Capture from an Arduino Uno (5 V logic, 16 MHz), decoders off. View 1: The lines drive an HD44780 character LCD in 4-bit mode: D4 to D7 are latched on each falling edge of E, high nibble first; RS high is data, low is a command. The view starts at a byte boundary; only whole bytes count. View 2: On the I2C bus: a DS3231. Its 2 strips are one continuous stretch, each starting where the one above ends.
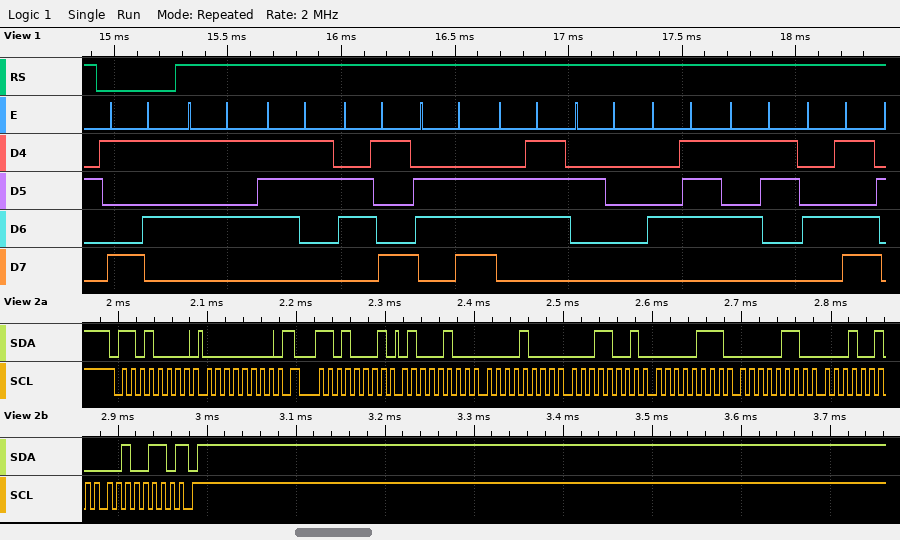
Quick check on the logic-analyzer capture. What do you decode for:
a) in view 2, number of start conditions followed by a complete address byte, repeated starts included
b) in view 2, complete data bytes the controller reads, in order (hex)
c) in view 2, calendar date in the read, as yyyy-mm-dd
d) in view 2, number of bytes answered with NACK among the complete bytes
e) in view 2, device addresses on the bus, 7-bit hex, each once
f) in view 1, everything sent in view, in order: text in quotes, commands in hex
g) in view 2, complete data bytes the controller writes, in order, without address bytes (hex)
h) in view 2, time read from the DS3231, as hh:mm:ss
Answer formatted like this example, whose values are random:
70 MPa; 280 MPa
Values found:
2; 44 08 19 07 06 12 26; 2026-12-06; 1; 0x68; 0x95 "Using GSM"; 00; 19:08:44
